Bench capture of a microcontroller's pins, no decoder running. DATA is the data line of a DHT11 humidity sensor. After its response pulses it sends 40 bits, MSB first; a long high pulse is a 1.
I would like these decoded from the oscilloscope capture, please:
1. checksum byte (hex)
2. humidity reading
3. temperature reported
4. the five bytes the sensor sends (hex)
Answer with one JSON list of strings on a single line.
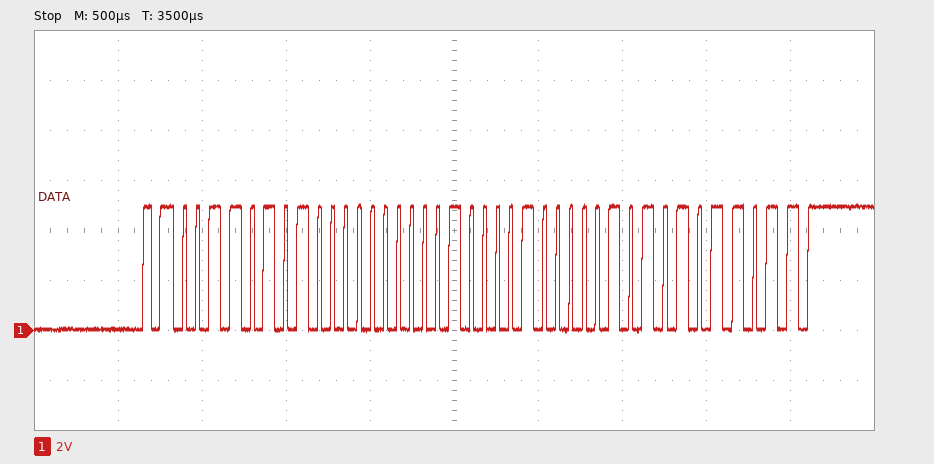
["0x5B", "53 %", "33.5 °C", "35 00 21 05 5B"]
